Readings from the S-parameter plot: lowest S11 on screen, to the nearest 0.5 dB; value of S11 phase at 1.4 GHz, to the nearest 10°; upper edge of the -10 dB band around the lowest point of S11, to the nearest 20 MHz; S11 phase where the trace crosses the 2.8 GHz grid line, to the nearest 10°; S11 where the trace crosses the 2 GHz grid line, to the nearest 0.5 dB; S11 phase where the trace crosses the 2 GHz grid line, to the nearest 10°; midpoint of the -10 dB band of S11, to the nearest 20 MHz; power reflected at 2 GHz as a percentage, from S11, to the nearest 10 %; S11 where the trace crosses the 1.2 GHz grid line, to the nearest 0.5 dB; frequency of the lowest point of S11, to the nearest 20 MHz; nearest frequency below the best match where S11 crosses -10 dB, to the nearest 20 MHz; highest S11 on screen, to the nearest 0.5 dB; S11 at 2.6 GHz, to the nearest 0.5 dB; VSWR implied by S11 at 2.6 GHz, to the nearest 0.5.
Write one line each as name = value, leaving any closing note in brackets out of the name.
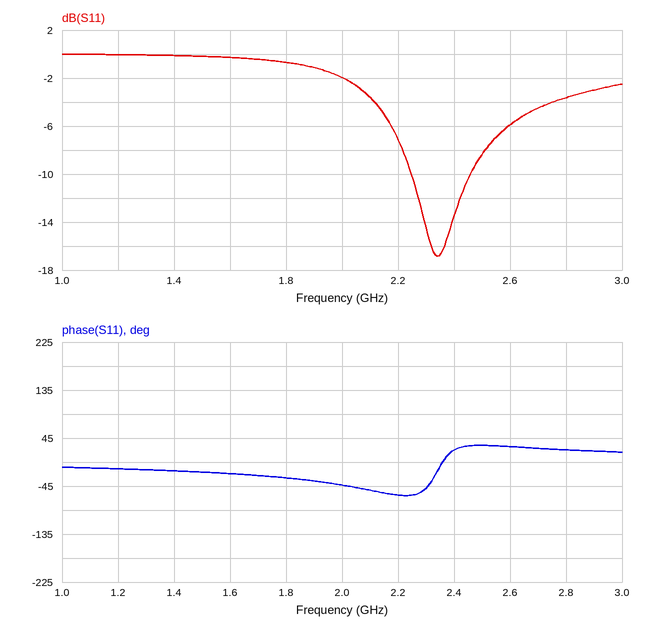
lowest S11 on screen, to the nearest 0.5 dB = -17.0 dB
value of S11 phase at 1.4 GHz, to the nearest 10° = -20°
upper edge of the -10 dB band around the lowest point of S11, to the nearest 20 MHz = 2.46 GHz
S11 phase where the trace crosses the 2.8 GHz grid line, to the nearest 10° = 20°
S11 where the trace crosses the 2 GHz grid line, to the nearest 0.5 dB = -2.0 dB
S11 phase where the trace crosses the 2 GHz grid line, to the nearest 10° = -40°
midpoint of the -10 dB band of S11, to the nearest 20 MHz = 2.36 GHz
power reflected at 2 GHz as a percentage, from S11, to the nearest 10 % = 60 %
S11 where the trace crosses the 1.2 GHz grid line, to the nearest 0.5 dB = 0.0 dB
frequency of the lowest point of S11, to the nearest 20 MHz = 2.34 GHz
nearest frequency below the best match where S11 crosses -10 dB, to the nearest 20 MHz = 2.24 GHz
highest S11 on screen, to the nearest 0.5 dB = 0.0 dB
S11 at 2.6 GHz, to the nearest 0.5 dB = -6.0 dB
VSWR implied by S11 at 2.6 GHz, to the nearest 0.5 = 3.0
